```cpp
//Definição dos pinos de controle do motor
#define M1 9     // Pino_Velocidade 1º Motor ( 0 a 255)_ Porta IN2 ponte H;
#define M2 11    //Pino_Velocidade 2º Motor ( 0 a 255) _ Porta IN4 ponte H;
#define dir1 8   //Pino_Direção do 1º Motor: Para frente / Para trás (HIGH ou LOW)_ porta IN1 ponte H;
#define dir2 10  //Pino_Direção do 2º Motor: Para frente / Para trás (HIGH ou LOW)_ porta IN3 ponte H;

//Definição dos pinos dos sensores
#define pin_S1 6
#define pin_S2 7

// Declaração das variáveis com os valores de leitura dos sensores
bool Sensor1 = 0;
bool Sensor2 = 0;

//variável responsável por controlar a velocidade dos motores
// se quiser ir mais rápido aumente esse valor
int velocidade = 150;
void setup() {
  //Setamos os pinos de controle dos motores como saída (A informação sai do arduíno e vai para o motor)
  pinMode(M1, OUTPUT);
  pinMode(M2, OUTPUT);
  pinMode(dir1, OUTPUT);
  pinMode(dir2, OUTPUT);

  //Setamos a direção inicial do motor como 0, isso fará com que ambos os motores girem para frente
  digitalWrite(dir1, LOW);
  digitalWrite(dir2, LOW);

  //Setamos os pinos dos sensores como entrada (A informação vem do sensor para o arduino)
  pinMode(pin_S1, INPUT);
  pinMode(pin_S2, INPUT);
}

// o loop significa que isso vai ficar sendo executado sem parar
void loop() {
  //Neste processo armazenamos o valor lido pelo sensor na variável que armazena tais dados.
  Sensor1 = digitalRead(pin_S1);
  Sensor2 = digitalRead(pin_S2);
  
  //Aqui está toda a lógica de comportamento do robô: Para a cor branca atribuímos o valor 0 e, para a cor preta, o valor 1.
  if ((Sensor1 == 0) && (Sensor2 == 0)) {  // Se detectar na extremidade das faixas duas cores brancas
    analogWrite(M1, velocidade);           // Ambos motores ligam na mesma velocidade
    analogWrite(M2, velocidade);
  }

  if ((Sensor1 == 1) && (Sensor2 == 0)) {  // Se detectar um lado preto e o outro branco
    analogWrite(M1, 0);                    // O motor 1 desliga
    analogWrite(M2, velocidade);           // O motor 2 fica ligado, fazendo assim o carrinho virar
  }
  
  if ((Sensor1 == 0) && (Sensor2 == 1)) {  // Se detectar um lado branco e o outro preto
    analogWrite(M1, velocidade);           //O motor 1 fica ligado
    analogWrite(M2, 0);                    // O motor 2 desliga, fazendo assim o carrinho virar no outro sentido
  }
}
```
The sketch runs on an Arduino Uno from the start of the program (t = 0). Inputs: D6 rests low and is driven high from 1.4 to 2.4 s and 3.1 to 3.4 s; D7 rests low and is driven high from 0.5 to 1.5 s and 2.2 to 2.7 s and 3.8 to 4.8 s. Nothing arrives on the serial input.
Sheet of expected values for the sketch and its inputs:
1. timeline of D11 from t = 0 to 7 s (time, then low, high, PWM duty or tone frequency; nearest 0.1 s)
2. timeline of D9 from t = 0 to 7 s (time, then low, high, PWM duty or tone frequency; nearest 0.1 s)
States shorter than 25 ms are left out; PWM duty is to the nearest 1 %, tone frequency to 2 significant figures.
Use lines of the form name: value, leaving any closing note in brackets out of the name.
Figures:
timeline of D11 from t = 0 to 7 s: 0 s PWM 59 %; 0.5 s low; 1.5 s PWM 59 %; 2.4 s low; 2.7 s PWM 59 %; 3.8 s low; 4.8 s PWM 59 %
timeline of D9 from t = 0 to 7 s: 0 s PWM 59 %; 1.5 s low; 2.4 s PWM 59 %; 3.1 s low; 3.4 s PWM 59 %
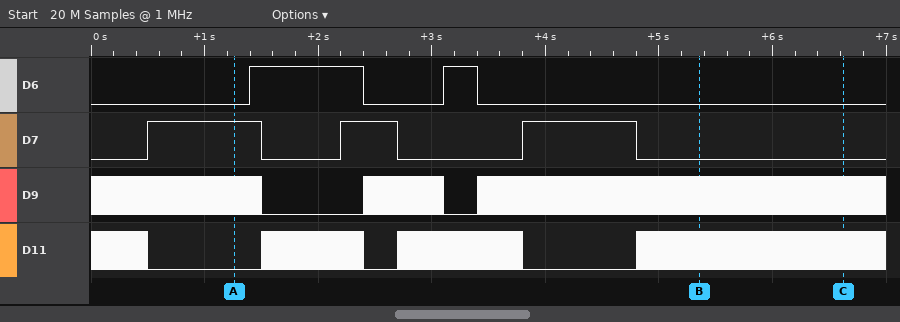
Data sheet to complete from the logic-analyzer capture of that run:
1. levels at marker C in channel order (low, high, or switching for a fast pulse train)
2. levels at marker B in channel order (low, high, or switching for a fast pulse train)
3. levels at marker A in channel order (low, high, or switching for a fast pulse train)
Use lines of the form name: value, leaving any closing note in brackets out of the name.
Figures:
levels at marker C in channel order: D6 low, D7 low, D9 switching, D11 switching
levels at marker B in channel order: D6 low, D7 low, D9 switching, D11 switching
levels at marker A in channel order: D6 low, D7 high, D9 switching, D11 low
